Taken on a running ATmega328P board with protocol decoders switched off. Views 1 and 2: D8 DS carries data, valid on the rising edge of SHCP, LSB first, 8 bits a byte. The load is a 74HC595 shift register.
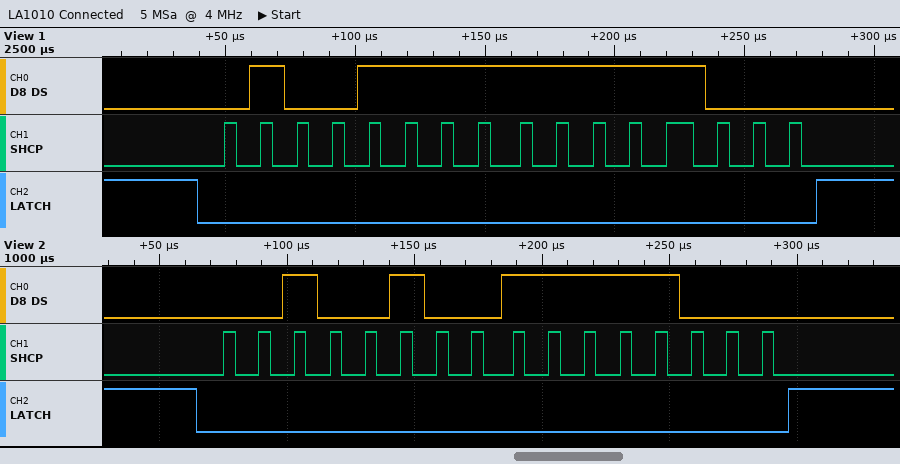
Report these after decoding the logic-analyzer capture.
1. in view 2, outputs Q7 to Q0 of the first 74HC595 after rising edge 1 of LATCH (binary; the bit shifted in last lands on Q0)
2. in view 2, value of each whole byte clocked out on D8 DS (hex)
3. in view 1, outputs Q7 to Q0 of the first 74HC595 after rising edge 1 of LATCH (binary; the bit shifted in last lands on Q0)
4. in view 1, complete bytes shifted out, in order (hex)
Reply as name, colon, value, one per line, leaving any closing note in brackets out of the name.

in view 2, outputs Q7 to Q0 of the first 74HC595 after rising edge 1 of LATCH: 11111000
in view 2, value of each whole byte clocked out on D8 DS: 24 1F
in view 1, outputs Q7 to Q0 of the first 74HC595 after rising edge 1 of LATCH: 11111000
in view 1, complete bytes shifted out, in order: 0xF2 0x1F
